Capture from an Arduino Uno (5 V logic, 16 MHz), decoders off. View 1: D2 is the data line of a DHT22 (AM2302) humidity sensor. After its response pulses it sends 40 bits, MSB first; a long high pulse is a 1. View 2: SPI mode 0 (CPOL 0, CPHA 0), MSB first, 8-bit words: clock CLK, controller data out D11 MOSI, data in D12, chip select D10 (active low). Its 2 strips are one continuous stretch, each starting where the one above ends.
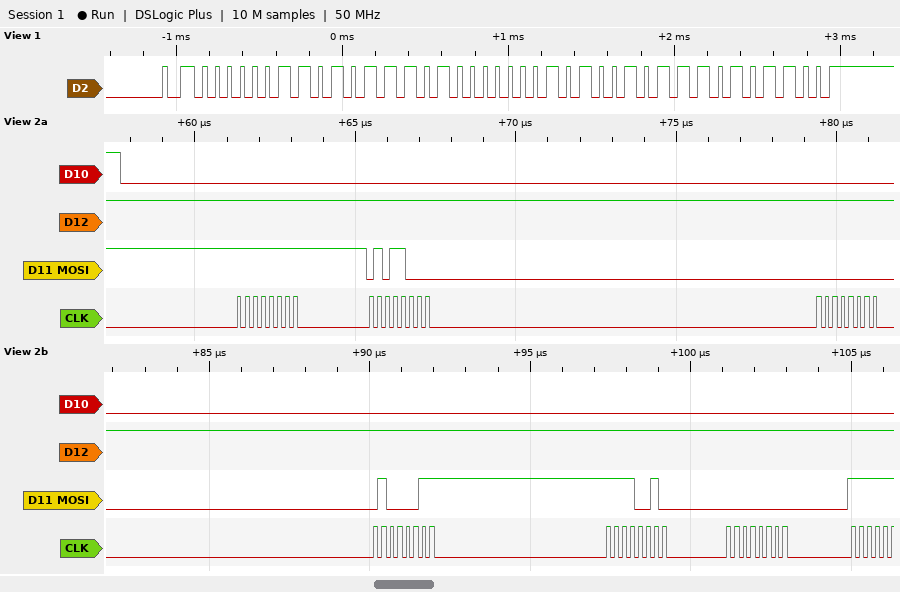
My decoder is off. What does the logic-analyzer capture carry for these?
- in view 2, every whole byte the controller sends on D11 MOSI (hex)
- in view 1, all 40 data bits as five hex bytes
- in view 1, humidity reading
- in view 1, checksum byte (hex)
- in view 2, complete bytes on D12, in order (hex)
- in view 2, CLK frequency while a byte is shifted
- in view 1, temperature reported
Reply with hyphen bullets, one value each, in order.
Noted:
- 0xFF 0x58 0x00 0x43 0xF2 0x00
- 03 5D 01 4B AC
- 86.1 %
- 0xAC
- 0xFF 0xFF 0xFF 0xFF 0xFF 0xFF
- 4 MHz
- 33.1 °C
